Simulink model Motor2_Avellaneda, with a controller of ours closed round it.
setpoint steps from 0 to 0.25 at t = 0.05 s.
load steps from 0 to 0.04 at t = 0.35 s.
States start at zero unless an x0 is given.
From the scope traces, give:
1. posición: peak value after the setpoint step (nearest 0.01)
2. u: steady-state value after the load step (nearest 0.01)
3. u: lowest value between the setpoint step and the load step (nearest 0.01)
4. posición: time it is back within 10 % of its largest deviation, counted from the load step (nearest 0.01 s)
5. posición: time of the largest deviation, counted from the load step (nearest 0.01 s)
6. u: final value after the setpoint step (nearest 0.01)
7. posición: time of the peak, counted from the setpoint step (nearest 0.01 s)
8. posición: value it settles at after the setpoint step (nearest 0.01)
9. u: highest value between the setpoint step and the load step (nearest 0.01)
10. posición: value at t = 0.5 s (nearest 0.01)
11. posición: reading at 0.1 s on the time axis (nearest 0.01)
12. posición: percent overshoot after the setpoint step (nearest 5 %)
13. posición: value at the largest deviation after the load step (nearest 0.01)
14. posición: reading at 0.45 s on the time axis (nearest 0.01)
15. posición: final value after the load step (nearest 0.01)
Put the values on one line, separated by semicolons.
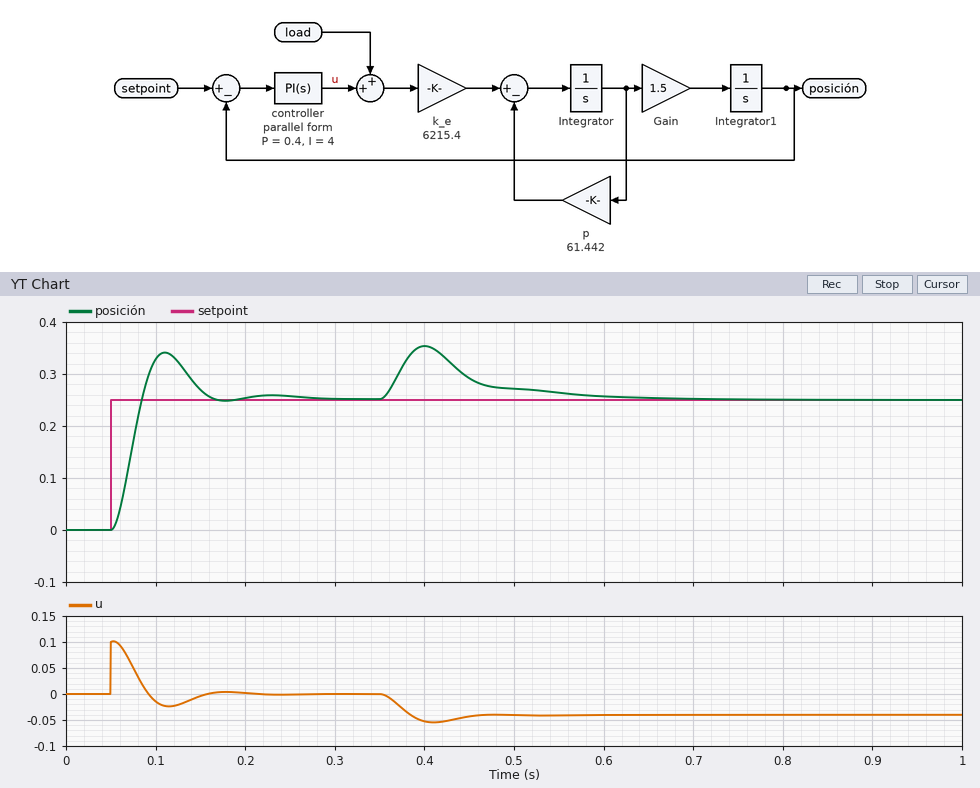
0.34; -0.04; -0.02; 0.22 s; 0.05 s; 0.00; 0.06 s; 0.25; 0.10; 0.27; 0.33; 35 %; 0.35; 0.29; 0.25
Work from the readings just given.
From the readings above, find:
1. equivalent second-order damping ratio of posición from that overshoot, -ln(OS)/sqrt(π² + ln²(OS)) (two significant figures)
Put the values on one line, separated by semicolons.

0.32
